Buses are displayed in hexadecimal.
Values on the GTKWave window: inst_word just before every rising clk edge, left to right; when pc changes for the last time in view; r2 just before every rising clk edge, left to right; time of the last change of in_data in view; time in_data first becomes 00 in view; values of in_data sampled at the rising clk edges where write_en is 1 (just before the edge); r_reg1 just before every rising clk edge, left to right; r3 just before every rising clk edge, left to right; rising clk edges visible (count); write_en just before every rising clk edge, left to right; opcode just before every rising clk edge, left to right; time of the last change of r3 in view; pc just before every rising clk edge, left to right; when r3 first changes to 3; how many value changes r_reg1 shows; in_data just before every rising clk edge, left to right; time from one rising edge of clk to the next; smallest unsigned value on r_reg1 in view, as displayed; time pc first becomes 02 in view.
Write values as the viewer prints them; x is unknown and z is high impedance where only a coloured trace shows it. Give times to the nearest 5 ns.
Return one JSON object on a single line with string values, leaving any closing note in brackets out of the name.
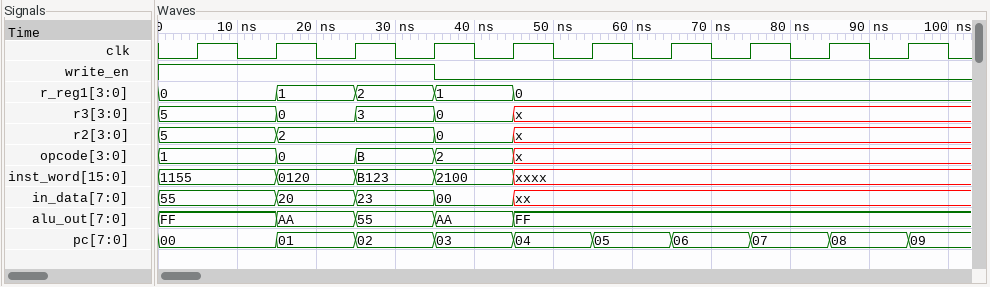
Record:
{"inst_word just before every rising clk edge, left to right": "1155, 1155, 0120, B123, 2100, xxxx, xxxx, xxxx, xxxx, xxxx", "when pc changes for the last time in view": "95 ns", "r2 just before every rising clk edge, left to right": "5, 5, 2, 2, 0, x, x, x, x, x", "time of the last change of in_data in view": "45 ns", "time in_data first becomes 00 in view": "35 ns", "values of in_data sampled at the rising clk edges where write_en is 1": "55, 55, 20, 23", "r_reg1 just before every rising clk edge, left to right": "0, 0, 1, 2, 1, 0, 0, 0, 0, 0", "r3 just before every rising clk edge, left to right": "5, 5, 0, 3, 0, x, x, x, x, x", "rising clk edges visible": "10", "write_en just before every rising clk edge, left to right": "1 1 1 1 0 0 0 0 0 0", "opcode just before every rising clk edge, left to right": "1, 1, 0, B, 2, x, x, x, x, x", "time of the last change of r3 in view": "45 ns", "pc just before every rising clk edge, left to right": "00, 00, 01, 02, 03, 04, 05, 06, 07, 08", "when r3 first changes to 3": "25 ns", "how many value changes r_reg1 shows": "4", "in_data just before every rising clk edge, left to right": "55, 55, 20, 23, 00, xx, xx, xx, xx, xx", "time from one rising edge of clk to the next": "10 ns", "smallest unsigned value on r_reg1 in view, as displayed": "0", "time pc first becomes 02 in view": "25 ns"}
